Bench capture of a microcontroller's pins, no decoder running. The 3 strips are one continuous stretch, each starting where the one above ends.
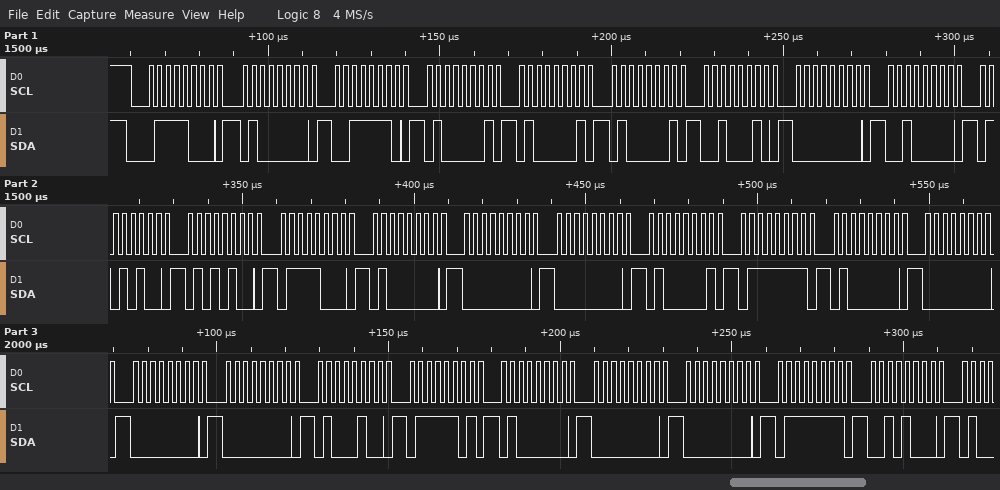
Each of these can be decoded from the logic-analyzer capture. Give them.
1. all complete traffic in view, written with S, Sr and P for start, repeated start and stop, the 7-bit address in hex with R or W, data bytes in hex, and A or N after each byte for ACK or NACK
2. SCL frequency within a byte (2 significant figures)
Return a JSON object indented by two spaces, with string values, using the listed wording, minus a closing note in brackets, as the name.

{
  "all complete traffic in view, written with S, Sr and P for start, repeated start and stop, the 7-bit address in hex with R or W, data bytes in hex, and A or N after each byte for ACK or NACK": "S 3CW A 40 A 3E A 41 A 41 A 41 A 22 A 00 A 20 A 54 A 54 A 78 A 40 A 00 A 00 A 41 A 7F A 40 A 00 A 00 A 00 A 44 A 7D A 40 A 00 A 00 A 7F A 28 A",
  "SCL frequency within a byte": "400 kHz"
}
